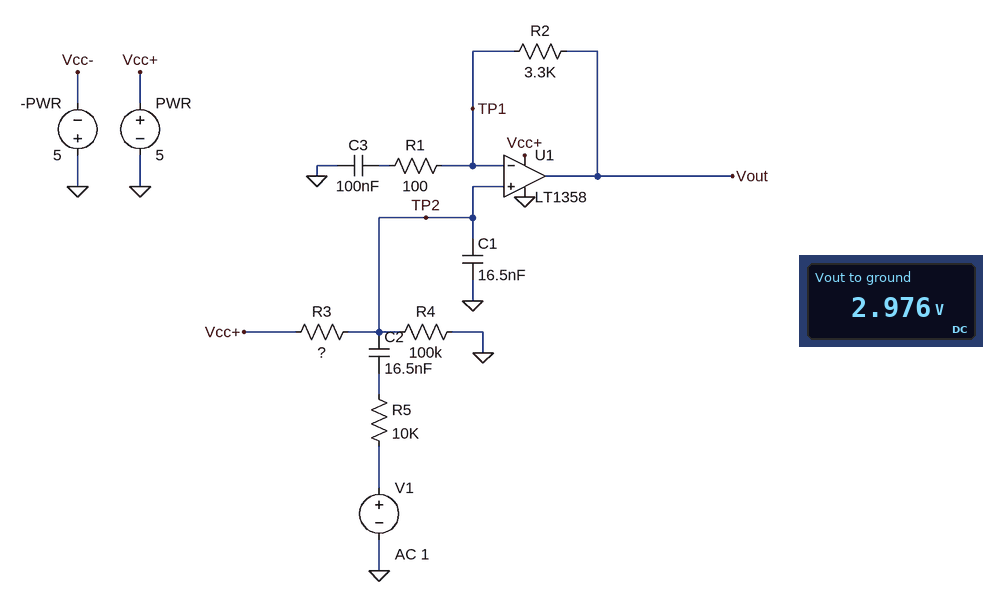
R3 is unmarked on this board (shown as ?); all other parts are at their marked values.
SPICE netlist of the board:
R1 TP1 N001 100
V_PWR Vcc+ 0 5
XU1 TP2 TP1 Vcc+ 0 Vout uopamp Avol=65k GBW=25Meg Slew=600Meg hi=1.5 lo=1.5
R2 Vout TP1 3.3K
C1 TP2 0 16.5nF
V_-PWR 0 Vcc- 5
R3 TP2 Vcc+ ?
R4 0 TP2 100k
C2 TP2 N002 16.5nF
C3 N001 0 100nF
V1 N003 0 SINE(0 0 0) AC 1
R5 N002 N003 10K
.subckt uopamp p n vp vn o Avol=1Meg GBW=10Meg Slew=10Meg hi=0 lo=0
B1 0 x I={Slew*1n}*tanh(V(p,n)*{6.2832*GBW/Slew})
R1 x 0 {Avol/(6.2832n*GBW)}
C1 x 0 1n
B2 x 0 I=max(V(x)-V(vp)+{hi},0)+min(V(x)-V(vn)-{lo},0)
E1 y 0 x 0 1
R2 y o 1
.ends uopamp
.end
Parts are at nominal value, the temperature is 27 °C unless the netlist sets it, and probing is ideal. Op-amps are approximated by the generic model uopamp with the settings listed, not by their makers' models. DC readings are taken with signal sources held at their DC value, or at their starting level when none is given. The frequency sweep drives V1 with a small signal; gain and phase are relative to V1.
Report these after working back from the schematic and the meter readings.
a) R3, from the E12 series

68 kΩ
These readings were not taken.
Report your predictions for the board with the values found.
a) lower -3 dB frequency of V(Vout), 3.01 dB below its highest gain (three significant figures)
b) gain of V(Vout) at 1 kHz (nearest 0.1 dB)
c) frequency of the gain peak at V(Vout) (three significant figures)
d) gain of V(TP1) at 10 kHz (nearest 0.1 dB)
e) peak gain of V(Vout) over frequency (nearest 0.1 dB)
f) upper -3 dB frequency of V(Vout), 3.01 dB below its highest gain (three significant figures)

1.57 kHz
-0.1 dB
5.69 kHz
-20.4 dB
5.3 dB
19.9 kHz
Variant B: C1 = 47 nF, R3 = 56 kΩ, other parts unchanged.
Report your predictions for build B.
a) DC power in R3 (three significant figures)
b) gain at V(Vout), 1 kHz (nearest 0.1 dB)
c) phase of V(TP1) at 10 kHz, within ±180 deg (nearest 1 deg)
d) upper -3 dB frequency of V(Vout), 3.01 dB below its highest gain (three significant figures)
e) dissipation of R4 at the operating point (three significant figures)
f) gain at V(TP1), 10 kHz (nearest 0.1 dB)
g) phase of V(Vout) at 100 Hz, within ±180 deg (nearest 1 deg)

57.5 µW
-6.4 dB
-82 deg
18.6 kHz
103 µW
-29.4 dB
42 deg
